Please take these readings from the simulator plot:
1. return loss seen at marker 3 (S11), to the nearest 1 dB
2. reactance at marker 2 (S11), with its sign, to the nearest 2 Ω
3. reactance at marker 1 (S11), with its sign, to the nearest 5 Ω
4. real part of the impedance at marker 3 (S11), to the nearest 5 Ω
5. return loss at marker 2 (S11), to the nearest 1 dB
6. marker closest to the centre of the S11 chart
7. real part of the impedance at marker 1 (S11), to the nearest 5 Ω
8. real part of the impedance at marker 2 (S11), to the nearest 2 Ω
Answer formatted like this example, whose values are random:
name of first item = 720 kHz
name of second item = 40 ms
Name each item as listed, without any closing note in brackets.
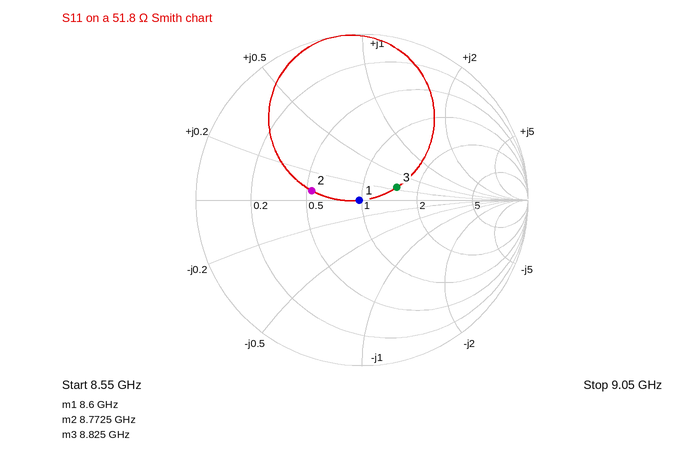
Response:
return loss seen at marker 3 (S11), to the nearest 1 dB = 13 dB
reactance at marker 2 (S11), with its sign, to the nearest 2 Ω = +4 Ω
reactance at marker 1 (S11), with its sign, to the nearest 5 Ω = 0 Ω
real part of the impedance at marker 3 (S11), to the nearest 5 Ω = 80 Ω
return loss at marker 2 (S11), to the nearest 1 dB = 10 dB
marker closest to the centre of the S11 chart = marker 1
real part of the impedance at marker 1 (S11), to the nearest 5 Ω = 50 Ω
real part of the impedance at marker 2 (S11), to the nearest 2 Ω = 28 Ω
